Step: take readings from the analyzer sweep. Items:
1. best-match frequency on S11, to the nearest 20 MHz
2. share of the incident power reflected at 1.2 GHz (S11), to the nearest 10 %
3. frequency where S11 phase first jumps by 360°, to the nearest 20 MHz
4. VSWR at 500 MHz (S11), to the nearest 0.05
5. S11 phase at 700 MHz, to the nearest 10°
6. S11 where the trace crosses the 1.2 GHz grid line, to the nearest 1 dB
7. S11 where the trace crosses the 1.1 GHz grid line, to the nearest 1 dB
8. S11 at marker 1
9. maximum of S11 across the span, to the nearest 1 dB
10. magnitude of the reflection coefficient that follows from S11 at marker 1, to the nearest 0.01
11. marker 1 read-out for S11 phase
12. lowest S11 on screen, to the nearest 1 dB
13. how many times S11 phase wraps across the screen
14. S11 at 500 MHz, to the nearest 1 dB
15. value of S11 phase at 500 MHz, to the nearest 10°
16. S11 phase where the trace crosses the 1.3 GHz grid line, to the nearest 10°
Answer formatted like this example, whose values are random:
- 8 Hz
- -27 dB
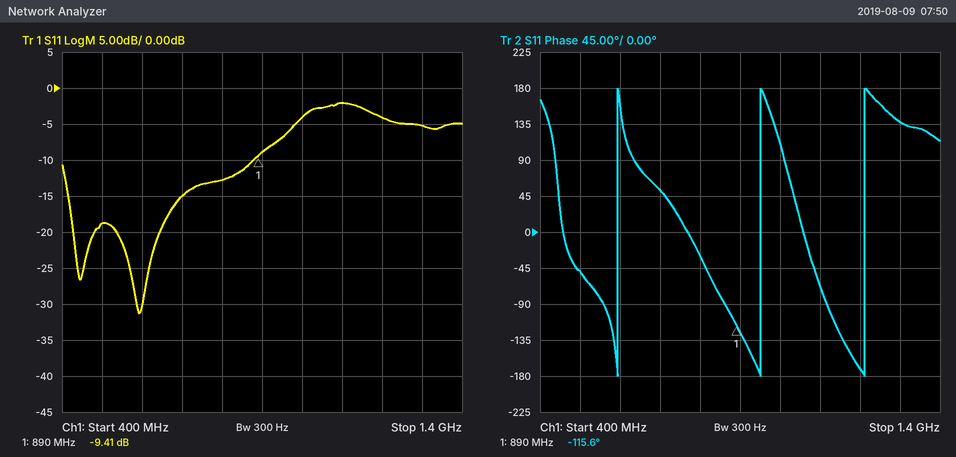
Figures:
- 600 MHz
- 40 %
- 600 MHz
- 1.25
- 50°
- -4 dB
- -2 dB
- -9.41 dB
- -2 dB
- 0.34
- -115.6°
- -31 dB
- 3
- -19 dB
- -50°
- 140°
